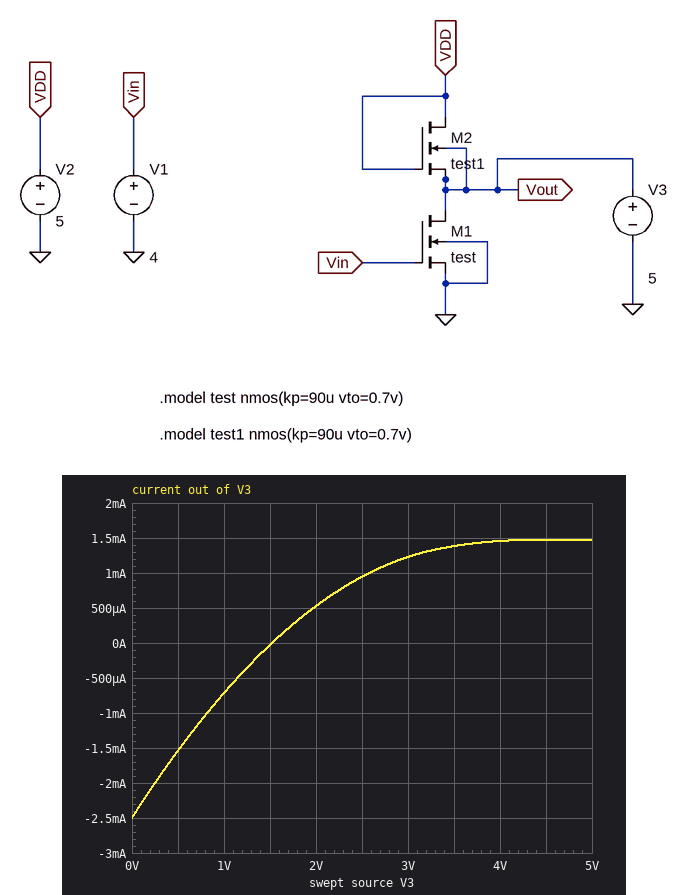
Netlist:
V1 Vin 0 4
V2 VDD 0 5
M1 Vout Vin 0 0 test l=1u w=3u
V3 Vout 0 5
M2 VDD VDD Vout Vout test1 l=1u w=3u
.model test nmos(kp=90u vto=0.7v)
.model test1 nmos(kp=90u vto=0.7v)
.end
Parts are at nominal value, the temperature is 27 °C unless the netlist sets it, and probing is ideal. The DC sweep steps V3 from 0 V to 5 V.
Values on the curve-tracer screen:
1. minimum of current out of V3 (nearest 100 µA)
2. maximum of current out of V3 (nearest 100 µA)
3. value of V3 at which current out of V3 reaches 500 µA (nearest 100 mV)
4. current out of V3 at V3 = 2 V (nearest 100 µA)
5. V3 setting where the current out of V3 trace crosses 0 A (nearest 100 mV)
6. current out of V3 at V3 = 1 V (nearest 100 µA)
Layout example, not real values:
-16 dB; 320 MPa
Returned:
-2.5 mA; 1.5 mA; 2.0 V; 500 µA; 1.5 V; -700 µA
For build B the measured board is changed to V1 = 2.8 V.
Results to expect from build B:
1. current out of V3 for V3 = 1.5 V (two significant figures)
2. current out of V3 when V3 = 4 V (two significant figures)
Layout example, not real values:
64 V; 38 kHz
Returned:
-510 µA; 580 µA
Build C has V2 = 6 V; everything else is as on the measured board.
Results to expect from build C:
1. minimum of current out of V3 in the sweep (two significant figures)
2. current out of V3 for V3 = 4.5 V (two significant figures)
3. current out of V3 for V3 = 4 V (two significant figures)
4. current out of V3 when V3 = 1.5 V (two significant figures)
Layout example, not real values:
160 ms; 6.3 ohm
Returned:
-3.8 mA; 1.4 mA; 1.2 mA; -920 µA
